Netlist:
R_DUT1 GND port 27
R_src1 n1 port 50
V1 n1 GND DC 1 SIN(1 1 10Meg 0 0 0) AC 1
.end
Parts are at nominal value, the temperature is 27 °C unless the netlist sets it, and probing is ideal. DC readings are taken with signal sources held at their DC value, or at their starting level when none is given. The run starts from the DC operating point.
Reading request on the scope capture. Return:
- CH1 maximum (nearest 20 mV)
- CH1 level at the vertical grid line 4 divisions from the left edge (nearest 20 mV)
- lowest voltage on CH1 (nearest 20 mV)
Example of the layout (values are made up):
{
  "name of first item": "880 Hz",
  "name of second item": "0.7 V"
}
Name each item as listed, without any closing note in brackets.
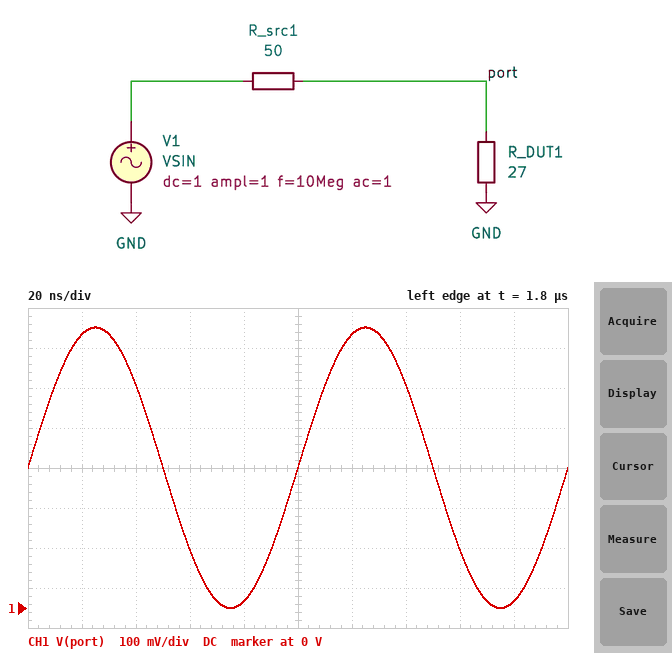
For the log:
{
  "CH1 maximum": "700 mV",
  "CH1 level at the vertical grid line 4 divisions from the left edge": "20 mV",
  "lowest voltage on CH1": "0 V"
}
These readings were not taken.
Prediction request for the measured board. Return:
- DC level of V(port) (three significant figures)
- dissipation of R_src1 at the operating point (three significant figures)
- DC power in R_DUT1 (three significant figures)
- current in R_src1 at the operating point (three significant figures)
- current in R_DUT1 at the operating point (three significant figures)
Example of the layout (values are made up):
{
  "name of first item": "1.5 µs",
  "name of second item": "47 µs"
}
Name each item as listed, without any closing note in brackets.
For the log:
{
  "DC level of V(port)": "351 mV",
  "dissipation of R_src1 at the operating point": "8.43 mW",
  "DC power in R_DUT1": "4.55 mW",
  "current in R_src1 at the operating point": "13.0 mA",
  "current in R_DUT1 at the operating point": "13.0 mA"
}
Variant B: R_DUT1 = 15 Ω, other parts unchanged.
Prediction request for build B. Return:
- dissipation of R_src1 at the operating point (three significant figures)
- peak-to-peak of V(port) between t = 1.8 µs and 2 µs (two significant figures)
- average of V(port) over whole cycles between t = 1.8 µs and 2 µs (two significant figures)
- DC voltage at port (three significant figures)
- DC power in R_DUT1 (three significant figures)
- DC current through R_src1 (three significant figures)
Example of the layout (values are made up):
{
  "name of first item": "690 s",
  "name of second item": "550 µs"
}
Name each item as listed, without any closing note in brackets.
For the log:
{
  "dissipation of R_src1 at the operating point": "11.8 mW",
  "peak-to-peak of V(port) between t = 1.8 µs and 2 µs": "460 mV",
  "average of V(port) over whole cycles between t = 1.8 µs and 2 µs": "230 mV",
  "DC voltage at port": "231 mV",
  "DC power in R_DUT1": "3.55 mW",
  "DC current through R_src1": "15.4 mA"
}
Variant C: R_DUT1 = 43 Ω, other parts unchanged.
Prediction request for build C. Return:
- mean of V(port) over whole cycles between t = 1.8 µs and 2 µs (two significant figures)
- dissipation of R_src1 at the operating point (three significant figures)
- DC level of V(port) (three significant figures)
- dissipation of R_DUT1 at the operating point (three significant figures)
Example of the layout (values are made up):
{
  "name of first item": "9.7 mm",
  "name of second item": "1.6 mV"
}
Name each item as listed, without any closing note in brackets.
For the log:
{
  "mean of V(port) over whole cycles between t = 1.8 µs and 2 µs": "460 mV",
  "dissipation of R_src1 at the operating point": "5.78 mW",
  "DC level of V(port)": "462 mV",
  "dissipation of R_DUT1 at the operating point": "4.97 mW"
}
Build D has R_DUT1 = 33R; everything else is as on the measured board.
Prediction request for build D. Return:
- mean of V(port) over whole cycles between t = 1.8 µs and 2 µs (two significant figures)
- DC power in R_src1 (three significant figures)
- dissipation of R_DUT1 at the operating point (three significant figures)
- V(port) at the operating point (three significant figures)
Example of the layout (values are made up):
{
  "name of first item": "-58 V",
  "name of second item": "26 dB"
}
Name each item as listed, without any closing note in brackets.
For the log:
{
  "mean of V(port) over whole cycles between t = 1.8 µs and 2 µs": "400 mV",
  "DC power in R_src1": "7.26 mW",
  "dissipation of R_DUT1 at the operating point": "4.79 mW",
  "V(port) at the operating point": "398 mV"
}
